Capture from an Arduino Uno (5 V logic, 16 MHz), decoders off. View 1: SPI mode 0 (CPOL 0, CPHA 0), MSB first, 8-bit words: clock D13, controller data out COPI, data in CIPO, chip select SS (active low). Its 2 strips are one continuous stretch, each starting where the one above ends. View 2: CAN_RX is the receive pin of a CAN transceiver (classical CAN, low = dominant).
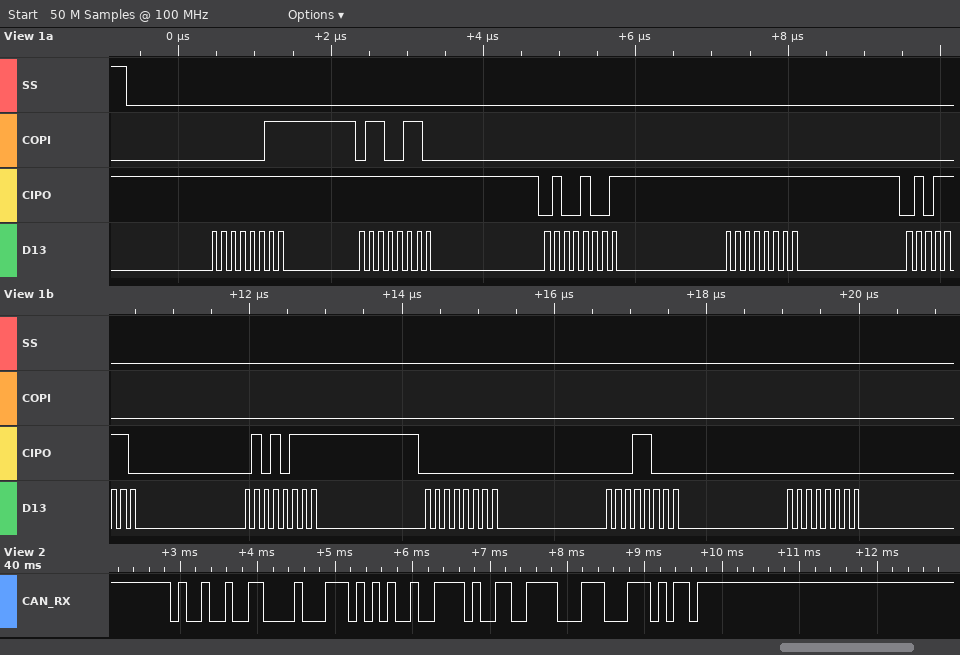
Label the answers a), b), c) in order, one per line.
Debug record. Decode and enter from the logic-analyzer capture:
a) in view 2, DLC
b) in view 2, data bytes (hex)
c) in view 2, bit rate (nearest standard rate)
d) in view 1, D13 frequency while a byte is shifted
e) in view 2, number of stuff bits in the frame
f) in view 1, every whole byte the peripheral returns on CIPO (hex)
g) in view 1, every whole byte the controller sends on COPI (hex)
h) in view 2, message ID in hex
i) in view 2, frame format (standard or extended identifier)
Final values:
a) 4
b) 75 49 E9 9E
c) 10 kbit/s
d) 8 MHz
e) 0
f) FF FF 49 FF 5E 57 00 18 00
g) 03 66 00 00 00 00 00 00 00
h) 0x493
i) standard
